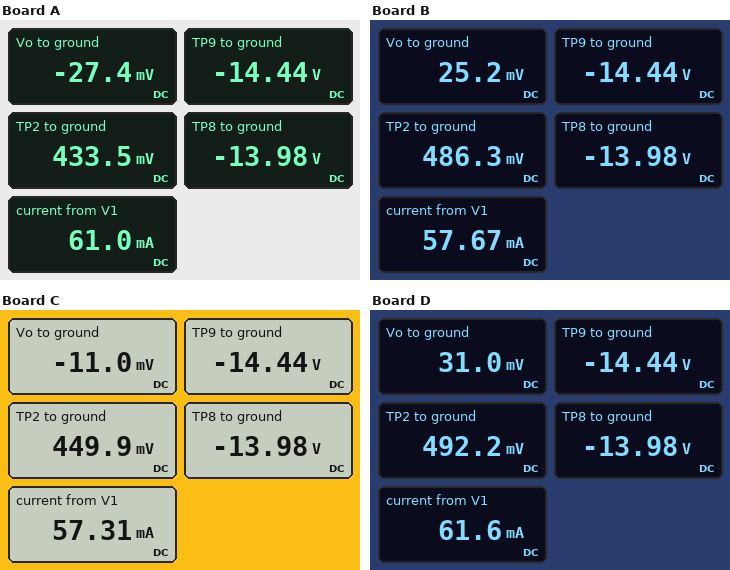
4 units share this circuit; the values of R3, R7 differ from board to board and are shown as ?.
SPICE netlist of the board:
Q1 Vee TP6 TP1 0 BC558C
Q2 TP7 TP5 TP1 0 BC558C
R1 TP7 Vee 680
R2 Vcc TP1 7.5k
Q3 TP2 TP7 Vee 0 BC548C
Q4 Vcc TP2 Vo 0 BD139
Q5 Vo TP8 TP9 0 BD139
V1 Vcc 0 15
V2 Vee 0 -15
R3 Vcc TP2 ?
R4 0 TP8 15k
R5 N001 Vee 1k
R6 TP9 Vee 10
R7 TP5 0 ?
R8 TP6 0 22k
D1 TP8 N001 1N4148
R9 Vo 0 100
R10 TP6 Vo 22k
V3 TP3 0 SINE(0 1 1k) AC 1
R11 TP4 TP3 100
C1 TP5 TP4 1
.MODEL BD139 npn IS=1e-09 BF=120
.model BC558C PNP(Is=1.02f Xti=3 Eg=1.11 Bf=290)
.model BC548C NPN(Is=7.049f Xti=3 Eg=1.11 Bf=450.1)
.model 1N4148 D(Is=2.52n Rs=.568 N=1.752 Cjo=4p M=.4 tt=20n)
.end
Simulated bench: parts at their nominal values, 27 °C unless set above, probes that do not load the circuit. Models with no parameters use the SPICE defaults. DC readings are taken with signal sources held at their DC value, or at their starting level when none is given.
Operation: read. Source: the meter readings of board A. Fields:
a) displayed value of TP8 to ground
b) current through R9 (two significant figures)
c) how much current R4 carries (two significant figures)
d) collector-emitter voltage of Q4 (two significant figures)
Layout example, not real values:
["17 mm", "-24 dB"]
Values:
["-13.98 V", "270 µA", "930 µA", "15 V"]
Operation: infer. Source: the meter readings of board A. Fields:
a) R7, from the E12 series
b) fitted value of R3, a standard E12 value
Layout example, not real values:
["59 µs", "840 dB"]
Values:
["3.9 kΩ", "3.3 kΩ"]
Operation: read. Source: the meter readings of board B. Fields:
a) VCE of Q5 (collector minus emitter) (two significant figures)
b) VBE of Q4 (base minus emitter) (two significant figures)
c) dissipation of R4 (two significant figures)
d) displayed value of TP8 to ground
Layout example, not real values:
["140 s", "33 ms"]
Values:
["14 V", "460 mV", "13 mW", "-13.98 V"]
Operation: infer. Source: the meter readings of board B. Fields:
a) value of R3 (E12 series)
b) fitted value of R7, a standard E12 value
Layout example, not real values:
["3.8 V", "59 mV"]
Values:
["27 kΩ", "18 kΩ"]
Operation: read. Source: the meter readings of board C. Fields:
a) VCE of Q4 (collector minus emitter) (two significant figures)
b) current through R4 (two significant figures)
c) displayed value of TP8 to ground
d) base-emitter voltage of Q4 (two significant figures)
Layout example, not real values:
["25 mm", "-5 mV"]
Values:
["15 V", "930 µA", "-13.98 V", "460 mV"]
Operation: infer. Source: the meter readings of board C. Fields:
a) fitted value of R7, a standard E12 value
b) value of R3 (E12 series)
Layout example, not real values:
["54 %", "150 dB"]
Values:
["12 kΩ", "27 kΩ"]
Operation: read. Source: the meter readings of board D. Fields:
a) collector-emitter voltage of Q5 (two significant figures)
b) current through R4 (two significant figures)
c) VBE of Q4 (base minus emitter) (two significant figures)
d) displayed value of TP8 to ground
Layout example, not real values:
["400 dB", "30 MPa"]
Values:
["14 V", "930 µA", "460 mV", "-13.98 V"]
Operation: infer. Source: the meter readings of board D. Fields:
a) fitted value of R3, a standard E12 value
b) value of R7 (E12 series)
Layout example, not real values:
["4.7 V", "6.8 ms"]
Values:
["3.3 kΩ", "12 kΩ"]
